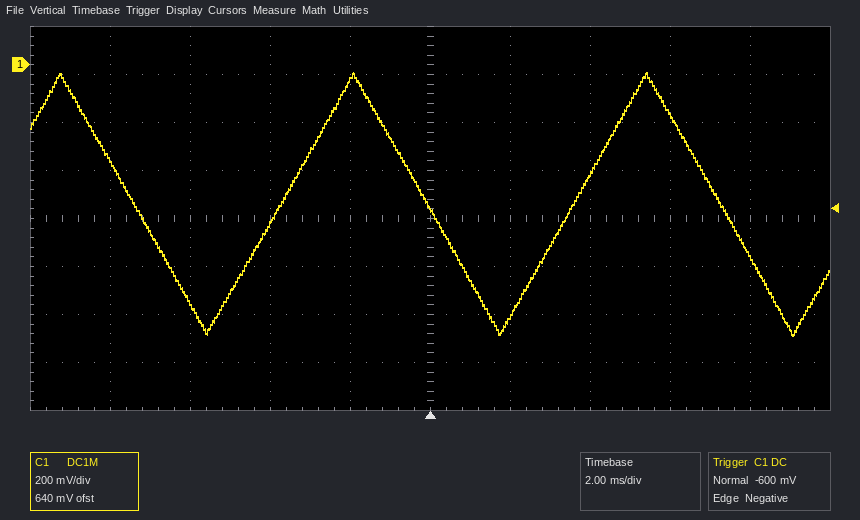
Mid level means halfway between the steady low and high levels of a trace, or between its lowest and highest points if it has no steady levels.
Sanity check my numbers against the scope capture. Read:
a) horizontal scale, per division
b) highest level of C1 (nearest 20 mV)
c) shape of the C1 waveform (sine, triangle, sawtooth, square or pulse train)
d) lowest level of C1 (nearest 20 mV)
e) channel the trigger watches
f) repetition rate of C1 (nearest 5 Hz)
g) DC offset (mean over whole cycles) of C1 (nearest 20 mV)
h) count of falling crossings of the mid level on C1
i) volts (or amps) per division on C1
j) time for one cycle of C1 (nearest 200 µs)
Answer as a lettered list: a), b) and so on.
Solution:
a) 2 ms
b) -40 mV
c) triangle
d) -1.12 V
e) C1
f) 135 Hz
g) -580 mV
h) 3
i) 200 mV
j) 7.4 ms
